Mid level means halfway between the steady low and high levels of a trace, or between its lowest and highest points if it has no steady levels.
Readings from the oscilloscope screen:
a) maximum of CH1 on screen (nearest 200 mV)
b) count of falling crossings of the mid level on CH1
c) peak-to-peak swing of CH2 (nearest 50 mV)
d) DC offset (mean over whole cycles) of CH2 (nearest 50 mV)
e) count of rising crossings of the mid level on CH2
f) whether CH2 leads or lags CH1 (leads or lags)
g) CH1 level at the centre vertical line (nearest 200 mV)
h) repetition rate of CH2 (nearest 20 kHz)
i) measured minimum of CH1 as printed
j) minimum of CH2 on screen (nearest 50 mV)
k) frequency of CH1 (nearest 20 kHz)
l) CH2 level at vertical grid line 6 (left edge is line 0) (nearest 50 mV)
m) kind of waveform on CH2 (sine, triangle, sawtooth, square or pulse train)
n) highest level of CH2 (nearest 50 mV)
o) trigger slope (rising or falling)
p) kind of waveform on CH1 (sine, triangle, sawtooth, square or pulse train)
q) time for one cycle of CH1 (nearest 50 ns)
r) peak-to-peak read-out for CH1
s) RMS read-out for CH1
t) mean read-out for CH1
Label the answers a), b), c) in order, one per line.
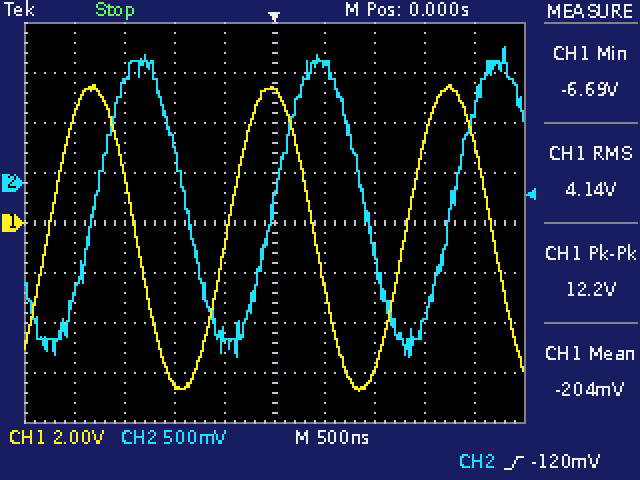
a) 5.6 V
b) 3
c) 3.10 V
d) -200 mV
e) 3
f) lags
g) 5.4 V
h) 560 kHz
i) -6.69 V
j) -1.75 V
k) 560 kHz
l) 1.20 V
m) sine
n) 1.35 V
o) rising
p) sine
q) 1.80 µs
r) 12.2 V
s) 4.14 V
t) -204 mV
